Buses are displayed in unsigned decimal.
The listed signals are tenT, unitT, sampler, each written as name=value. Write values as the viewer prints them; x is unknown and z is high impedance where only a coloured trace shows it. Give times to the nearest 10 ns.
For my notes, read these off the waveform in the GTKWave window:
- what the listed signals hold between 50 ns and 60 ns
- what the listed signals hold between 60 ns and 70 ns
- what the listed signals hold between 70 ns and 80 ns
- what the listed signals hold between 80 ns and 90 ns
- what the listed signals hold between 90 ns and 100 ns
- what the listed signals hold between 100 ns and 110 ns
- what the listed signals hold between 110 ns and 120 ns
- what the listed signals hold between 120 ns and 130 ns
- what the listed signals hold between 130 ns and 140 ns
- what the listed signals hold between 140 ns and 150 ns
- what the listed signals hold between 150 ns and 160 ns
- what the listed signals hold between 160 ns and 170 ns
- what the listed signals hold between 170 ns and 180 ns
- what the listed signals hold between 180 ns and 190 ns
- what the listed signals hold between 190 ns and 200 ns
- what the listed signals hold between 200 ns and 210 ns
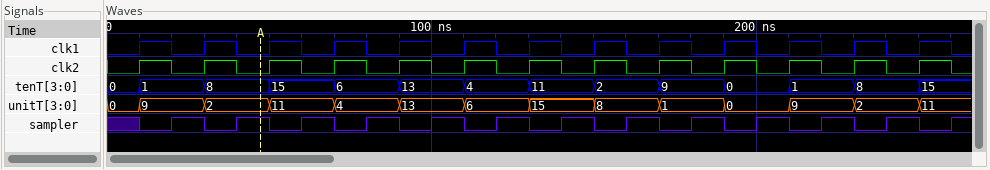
tenT=15, unitT=11, sampler=0
tenT=15, unitT=11, sampler=1
tenT=6, unitT=4, sampler=0
tenT=6, unitT=4, sampler=1
tenT=13, unitT=13, sampler=0
tenT=13, unitT=13, sampler=1
tenT=4, unitT=6, sampler=0
tenT=4, unitT=6, sampler=1
tenT=11, unitT=15, sampler=0
tenT=11, unitT=15, sampler=1
tenT=2, unitT=8, sampler=0
tenT=2, unitT=8, sampler=1
tenT=9, unitT=1, sampler=0
tenT=9, unitT=1, sampler=1
tenT=0, unitT=0, sampler=0
tenT=0, unitT=0, sampler=1
